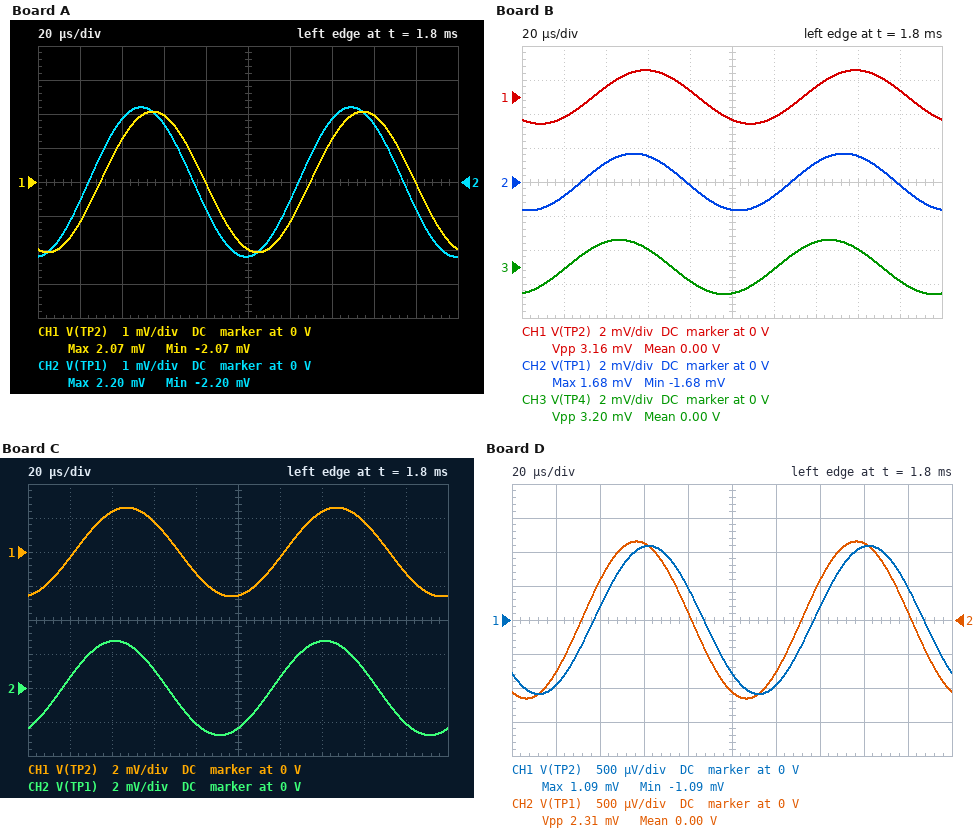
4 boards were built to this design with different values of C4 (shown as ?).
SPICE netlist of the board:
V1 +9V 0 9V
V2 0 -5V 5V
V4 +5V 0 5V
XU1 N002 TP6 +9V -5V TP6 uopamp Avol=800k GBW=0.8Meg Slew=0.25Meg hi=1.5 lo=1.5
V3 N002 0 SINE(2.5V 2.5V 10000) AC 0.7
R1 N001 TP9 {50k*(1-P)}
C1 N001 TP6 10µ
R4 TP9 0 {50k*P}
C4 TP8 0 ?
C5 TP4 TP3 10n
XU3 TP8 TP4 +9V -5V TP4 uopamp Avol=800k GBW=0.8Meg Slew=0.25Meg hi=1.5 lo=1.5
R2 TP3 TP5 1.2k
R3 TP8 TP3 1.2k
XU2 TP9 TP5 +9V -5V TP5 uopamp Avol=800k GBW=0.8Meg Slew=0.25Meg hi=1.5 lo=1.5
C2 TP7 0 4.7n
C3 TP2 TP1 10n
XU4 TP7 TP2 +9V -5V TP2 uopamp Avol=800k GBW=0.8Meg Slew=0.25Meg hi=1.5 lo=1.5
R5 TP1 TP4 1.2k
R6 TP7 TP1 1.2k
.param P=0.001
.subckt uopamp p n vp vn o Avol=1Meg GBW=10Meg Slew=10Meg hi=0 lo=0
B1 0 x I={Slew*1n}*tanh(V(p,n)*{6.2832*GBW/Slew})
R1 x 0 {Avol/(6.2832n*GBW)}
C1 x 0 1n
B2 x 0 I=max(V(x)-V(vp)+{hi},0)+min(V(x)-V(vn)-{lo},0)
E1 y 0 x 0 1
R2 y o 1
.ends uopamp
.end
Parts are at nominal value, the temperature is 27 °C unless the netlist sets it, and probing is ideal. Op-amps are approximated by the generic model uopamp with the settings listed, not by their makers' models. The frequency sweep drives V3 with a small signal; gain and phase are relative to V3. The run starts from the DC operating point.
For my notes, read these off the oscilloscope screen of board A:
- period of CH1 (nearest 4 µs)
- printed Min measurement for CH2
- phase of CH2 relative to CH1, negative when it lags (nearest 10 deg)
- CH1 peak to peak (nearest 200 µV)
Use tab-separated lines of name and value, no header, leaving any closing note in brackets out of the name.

period of CH1	100 µs
printed Min measurement for CH2	-2.20 mV
phase of CH2 relative to CH1, negative when it lags	20 deg
CH1 peak to peak	4.2 mV
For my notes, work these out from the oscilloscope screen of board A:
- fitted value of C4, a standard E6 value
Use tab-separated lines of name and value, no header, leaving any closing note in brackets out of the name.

fitted value of C4, a standard E6 value	6.8 nF
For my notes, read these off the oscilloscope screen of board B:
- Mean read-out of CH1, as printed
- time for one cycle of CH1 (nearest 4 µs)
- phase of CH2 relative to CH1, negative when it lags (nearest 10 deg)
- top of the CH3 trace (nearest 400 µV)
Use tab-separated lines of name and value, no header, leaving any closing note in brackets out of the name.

Mean read-out of CH1, as printed	0.00 V
time for one cycle of CH1	100 µs
phase of CH2 relative to CH1, negative when it lags	20 deg
top of the CH3 trace	1.6 mV
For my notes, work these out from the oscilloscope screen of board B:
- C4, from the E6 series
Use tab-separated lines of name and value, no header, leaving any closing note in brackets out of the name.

C4, from the E6 series	10 nF
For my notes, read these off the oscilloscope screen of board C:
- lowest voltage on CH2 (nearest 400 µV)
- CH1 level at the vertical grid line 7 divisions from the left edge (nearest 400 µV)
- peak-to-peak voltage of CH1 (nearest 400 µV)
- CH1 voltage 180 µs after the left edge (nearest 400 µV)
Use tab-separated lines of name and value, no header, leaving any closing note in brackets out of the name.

lowest voltage on CH2	-2.8 mV
CH1 level at the vertical grid line 7 divisions from the left edge	2.4 mV
peak-to-peak voltage of CH1	5.2 mV
CH1 voltage 180 µs after the left edge	-1.2 mV
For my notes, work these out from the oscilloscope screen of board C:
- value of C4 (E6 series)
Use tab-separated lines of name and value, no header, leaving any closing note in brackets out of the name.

value of C4	3.3 nF
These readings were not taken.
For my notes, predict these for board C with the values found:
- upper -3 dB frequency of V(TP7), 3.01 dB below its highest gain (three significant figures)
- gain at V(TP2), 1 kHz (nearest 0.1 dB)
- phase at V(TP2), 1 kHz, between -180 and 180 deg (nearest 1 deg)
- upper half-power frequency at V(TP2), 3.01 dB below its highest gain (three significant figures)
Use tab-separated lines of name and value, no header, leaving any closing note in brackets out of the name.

upper -3 dB frequency of V(TP7), 3.01 dB below its highest gain	19.2 kHz
gain at V(TP2), 1 kHz	-60.0 dB
phase at V(TP2), 1 kHz, between -180 and 180 deg	-7 deg
upper half-power frequency at V(TP2), 3.01 dB below its highest gain	19.2 kHz
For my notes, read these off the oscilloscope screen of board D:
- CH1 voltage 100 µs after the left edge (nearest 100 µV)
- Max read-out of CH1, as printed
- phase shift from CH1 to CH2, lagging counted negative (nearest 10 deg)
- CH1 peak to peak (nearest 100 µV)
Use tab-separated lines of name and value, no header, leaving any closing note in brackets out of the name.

CH1 voltage 100 µs after the left edge	-800 µV
Max read-out of CH1, as printed	1.09 mV
phase shift from CH1 to CH2, lagging counted negative	20 deg
CH1 peak to peak	2.2 mV
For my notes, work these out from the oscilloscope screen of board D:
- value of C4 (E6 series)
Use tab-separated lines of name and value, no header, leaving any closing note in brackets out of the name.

value of C4	15 nF
